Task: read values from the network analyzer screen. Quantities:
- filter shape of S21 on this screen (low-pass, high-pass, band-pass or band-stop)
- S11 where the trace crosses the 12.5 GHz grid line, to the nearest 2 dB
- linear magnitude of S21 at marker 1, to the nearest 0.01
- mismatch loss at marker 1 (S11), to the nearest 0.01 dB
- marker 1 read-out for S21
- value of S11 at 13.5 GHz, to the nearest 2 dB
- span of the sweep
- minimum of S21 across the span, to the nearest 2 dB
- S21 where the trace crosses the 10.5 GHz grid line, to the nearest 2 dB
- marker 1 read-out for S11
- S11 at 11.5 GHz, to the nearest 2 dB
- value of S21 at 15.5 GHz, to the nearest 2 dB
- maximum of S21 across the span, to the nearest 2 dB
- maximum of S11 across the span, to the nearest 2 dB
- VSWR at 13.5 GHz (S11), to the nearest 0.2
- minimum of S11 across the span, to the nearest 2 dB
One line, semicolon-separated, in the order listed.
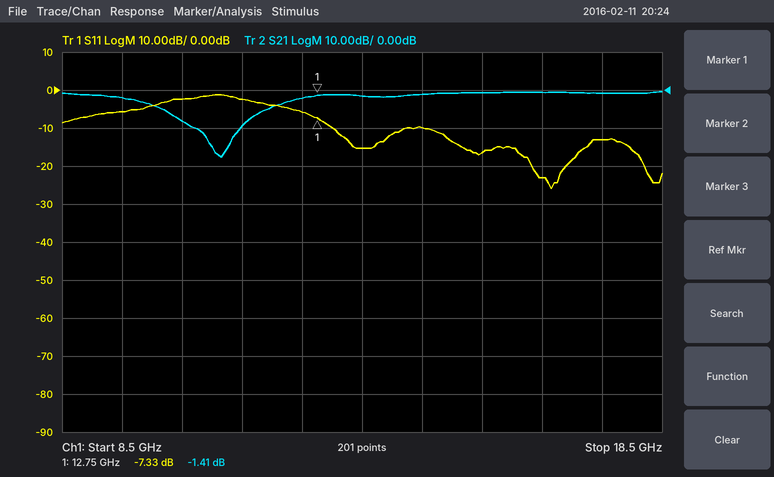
band-stop; -6 dB; 0.85; 0.89 dB; -1.41 dB; -16 dB; 10 GHz; -18 dB; -8 dB; -7.33 dB; -2 dB; 0 dB; 0 dB; -2 dB; 1.4; -26 dB
